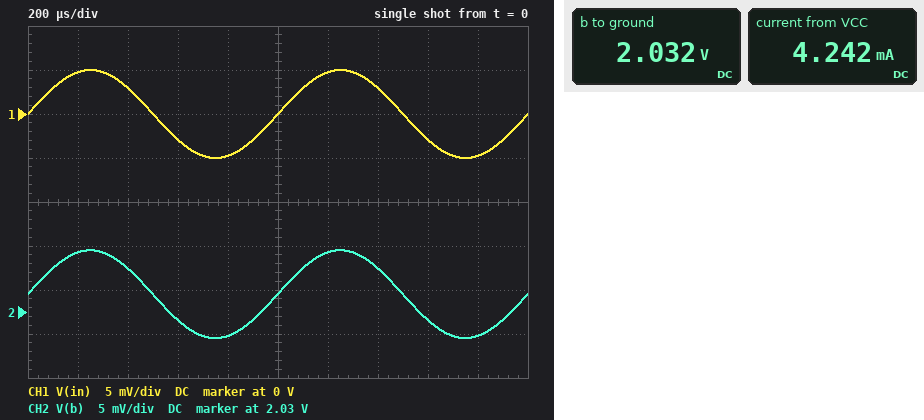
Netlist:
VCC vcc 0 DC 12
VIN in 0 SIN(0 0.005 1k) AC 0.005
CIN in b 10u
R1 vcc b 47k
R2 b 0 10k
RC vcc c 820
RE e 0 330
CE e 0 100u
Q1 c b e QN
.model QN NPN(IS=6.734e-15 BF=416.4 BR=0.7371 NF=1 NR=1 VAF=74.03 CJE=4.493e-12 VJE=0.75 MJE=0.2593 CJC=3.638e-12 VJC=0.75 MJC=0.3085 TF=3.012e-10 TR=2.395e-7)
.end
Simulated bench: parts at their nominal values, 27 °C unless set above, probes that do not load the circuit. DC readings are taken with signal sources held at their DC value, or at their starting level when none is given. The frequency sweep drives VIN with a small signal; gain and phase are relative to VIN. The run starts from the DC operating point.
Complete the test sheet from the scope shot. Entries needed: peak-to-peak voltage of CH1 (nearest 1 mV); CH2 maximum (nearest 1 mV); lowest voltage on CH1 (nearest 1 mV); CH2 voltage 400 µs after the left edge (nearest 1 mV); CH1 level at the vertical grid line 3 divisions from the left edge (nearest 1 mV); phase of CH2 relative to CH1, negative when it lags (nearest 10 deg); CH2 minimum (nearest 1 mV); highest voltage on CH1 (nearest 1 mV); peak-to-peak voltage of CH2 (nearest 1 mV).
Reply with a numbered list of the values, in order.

1. 10 mV
2. 2.037 V
3. -5 mV
4. 2.035 V
5. -3 mV
6. 0 deg
7. 2.027 V
8. 5 mV
9. 10 mV
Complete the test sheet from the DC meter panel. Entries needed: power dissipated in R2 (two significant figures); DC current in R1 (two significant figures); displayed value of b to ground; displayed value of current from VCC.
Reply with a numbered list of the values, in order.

1. 410 µW
2. 210 µA
3. 2.032 V
4. 4.242 mA
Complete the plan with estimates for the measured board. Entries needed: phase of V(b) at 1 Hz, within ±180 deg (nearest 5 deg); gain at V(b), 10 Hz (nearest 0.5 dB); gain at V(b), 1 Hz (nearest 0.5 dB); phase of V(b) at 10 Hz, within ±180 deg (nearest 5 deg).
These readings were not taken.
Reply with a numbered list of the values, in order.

1. 65 deg
2. -0.5 dB
3. -7.0 dB
4. 10 deg
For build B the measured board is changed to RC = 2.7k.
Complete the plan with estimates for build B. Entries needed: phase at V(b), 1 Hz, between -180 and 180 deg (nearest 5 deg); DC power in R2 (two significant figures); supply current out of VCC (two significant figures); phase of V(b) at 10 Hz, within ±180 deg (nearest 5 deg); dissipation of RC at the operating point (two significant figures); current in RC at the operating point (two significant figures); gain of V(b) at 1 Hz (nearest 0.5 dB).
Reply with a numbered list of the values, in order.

1. 80 deg
2. 400 µW
3. 4.1 mA
4. 25 deg
5. 41 mW
6. 3.9 mA
7. -25.5 dB
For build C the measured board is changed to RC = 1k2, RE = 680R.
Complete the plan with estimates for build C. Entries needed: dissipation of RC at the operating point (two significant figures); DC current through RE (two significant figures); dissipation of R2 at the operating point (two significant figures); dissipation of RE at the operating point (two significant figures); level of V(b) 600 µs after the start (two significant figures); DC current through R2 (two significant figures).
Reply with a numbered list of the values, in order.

1. 5.0 mW
2. 2.0 mA
3. 430 µW
4. 2.8 mW
5. 2.1 V
6. 210 µA
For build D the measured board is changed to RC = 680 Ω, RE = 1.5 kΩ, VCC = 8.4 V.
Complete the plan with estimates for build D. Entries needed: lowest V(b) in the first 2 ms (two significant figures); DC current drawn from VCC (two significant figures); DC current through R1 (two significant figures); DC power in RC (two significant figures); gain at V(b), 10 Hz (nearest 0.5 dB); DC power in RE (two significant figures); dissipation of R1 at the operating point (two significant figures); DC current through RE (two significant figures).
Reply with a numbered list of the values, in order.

1. 1.5 V
2. 690 µA
3. 150 µA
4. 200 µW
5. -0.5 dB
6. 440 µW
7. 1.0 mW
8. 540 µA
